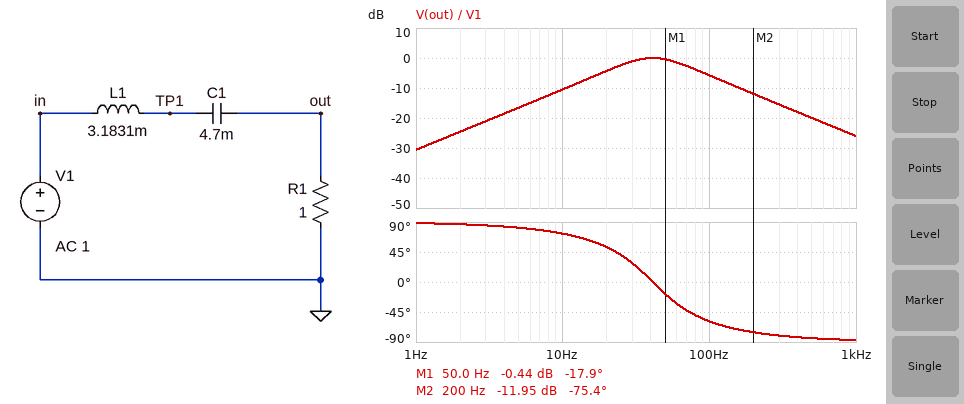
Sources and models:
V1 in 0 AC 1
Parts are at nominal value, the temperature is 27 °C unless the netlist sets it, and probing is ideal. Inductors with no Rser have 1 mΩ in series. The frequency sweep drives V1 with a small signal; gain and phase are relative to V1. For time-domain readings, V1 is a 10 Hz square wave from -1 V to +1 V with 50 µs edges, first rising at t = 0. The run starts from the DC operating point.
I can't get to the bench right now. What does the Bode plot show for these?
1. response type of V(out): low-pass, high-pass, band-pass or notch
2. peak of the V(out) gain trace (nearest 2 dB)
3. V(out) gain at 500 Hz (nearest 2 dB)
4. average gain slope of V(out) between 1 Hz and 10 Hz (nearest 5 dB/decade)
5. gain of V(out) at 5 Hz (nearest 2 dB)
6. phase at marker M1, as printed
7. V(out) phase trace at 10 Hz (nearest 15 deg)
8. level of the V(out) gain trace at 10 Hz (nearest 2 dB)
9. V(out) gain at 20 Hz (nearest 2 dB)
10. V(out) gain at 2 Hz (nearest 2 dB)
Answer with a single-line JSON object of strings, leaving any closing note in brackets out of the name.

{"response type of V(out): low-pass, high-pass, band-pass or notch": "band-pass", "peak of the V(out) gain trace": "0 dB", "V(out) gain at 500 Hz": "-20 dB", "average gain slope of V(out) between 1 Hz and 10 Hz": "20 dB/decade", "gain of V(out) at 5 Hz": "-16 dB", "phase at marker M1, as printed": "-17.9 deg", "V(out) phase trace at 10 Hz": "75 deg", "level of the V(out) gain trace at 10 Hz": "-10 dB", "V(out) gain at 20 Hz": "-4 dB", "V(out) gain at 2 Hz": "-24 dB"}
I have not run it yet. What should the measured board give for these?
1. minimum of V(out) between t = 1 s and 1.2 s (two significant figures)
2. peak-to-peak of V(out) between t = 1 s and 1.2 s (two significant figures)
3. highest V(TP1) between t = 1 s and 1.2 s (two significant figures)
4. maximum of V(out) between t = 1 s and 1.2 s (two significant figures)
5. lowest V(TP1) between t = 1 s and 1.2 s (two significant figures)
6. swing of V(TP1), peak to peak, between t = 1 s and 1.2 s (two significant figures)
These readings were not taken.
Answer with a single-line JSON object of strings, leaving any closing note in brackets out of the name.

{"minimum of V(out) between t = 1 s and 1.2 s": "-1.2 V", "peak-to-peak of V(out) between t = 1 s and 1.2 s": "2.4 V", "highest V(TP1) between t = 1 s and 1.2 s": "1.5 V", "maximum of V(out) between t = 1 s and 1.2 s": "1.2 V", "lowest V(TP1) between t = 1 s and 1.2 s": "-1.5 V", "swing of V(TP1), peak to peak, between t = 1 s and 1.2 s": "3.0 V"}
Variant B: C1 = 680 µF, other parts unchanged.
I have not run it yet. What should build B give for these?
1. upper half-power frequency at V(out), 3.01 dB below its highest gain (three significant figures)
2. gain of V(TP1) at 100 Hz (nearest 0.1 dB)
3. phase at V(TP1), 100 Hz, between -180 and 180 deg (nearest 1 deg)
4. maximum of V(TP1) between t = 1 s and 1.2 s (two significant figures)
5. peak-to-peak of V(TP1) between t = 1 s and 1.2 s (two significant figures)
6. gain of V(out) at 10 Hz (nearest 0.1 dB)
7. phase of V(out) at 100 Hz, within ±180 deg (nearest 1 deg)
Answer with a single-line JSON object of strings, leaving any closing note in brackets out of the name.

{"upper half-power frequency at V(out), 3.01 dB below its highest gain": "136 Hz", "gain of V(TP1) at 100 Hz": "7.6 dB", "phase at V(TP1), 100 Hz, between -180 and 180 deg": "-48 deg", "maximum of V(TP1) between t = 1 s and 1.2 s": "2.1 V", "peak-to-peak of V(TP1) between t = 1 s and 1.2 s": "4.1 V", "gain of V(out) at 10 Hz": "-27.3 dB", "phase of V(out) at 100 Hz, within ±180 deg": "19 deg"}
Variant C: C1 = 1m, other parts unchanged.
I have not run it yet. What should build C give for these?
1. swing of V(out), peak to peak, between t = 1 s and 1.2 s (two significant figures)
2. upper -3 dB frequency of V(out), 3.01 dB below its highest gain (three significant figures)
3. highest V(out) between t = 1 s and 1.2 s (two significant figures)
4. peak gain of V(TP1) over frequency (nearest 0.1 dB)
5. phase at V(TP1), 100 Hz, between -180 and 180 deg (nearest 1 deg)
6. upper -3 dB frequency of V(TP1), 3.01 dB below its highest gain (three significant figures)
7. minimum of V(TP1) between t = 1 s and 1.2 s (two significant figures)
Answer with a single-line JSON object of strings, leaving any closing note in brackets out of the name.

{"swing of V(out), peak to peak, between t = 1 s and 1.2 s": "1.5 V", "upper -3 dB frequency of V(out), 3.01 dB below its highest gain": "118 Hz", "highest V(out) between t = 1 s and 1.2 s": "770 mV", "peak gain of V(TP1) over frequency": "6.4 dB", "phase at V(TP1), 100 Hz, between -180 and 180 deg": "-80 deg", "upper -3 dB frequency of V(TP1), 3.01 dB below its highest gain": "108 Hz", "minimum of V(TP1) between t = 1 s and 1.2 s": "-1.9 V"}
